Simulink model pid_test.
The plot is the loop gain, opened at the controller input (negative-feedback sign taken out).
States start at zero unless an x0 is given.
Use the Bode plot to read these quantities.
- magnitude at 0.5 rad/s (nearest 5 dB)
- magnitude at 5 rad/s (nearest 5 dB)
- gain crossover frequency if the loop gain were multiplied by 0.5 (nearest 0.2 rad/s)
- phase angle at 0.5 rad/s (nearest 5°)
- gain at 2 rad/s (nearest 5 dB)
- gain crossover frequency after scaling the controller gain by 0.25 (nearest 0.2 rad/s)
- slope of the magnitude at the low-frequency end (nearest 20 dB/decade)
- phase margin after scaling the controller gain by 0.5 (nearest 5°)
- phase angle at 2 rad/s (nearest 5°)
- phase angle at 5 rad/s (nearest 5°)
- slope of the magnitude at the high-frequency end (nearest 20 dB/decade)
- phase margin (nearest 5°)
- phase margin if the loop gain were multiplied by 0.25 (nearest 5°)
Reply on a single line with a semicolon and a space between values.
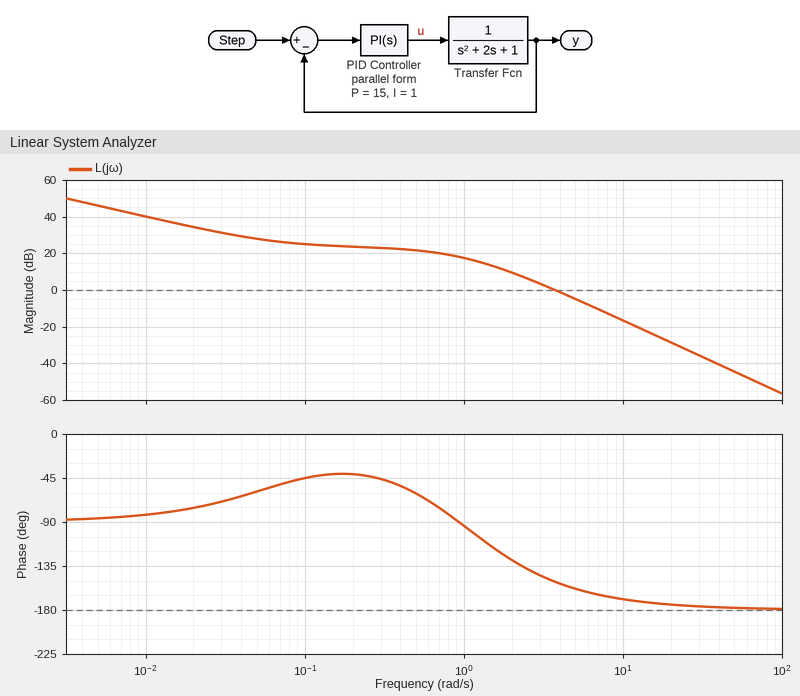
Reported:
20 dB; -5 dB; 2.6 rad/s; -60°; 10 dB; 1.6 rad/s; -20 dB/decade; 40°; -130°; -160°; -40 dB/decade; 30°; 60°
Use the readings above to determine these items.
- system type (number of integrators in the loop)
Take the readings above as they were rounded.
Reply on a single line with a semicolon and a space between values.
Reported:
1
